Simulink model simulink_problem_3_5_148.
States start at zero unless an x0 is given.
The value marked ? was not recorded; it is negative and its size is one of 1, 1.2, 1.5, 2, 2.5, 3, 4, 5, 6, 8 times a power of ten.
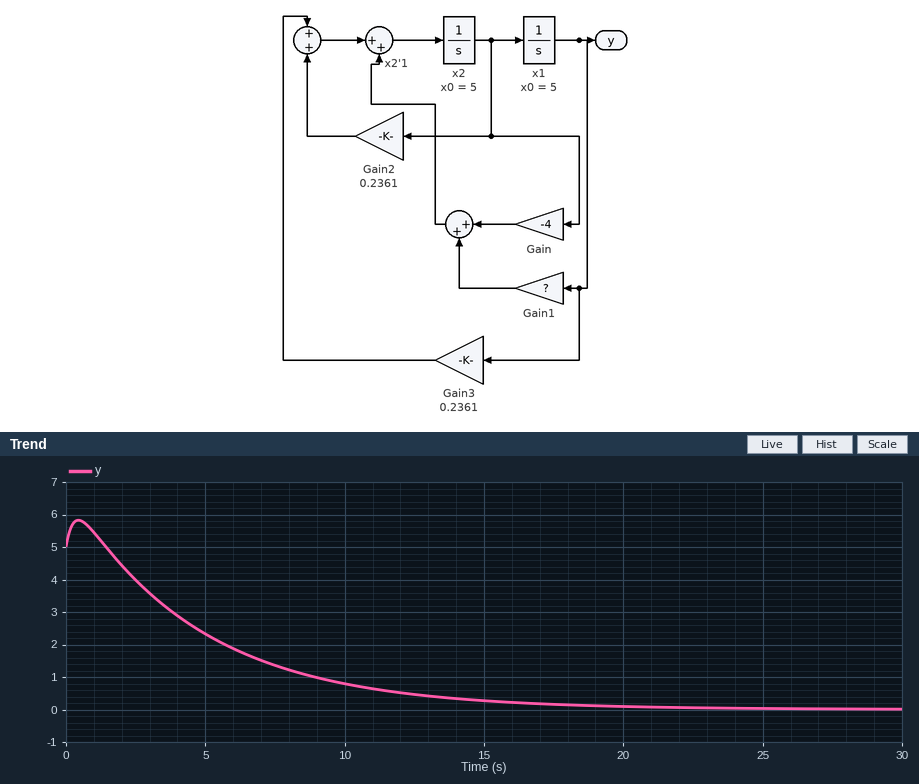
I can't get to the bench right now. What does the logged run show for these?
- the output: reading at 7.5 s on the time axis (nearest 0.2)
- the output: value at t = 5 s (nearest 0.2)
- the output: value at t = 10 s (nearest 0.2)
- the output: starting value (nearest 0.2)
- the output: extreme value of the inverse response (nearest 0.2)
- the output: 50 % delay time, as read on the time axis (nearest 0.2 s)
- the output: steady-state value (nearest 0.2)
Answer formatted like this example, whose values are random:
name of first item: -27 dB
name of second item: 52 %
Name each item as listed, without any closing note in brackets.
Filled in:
the output: reading at 7.5 s on the time axis: 1.4
the output: value at t = 5 s: 2.4
the output: value at t = 10 s: 0.8
the output: starting value: 5.0
the output: extreme value of the inverse response: 5.8
the output: 50 % delay time, as read on the time axis: 4.6 s
the output: steady-state value: 0.0
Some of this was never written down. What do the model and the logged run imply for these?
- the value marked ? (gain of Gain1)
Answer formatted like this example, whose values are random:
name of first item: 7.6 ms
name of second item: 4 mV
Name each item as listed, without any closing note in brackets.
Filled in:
the value marked ?: -1
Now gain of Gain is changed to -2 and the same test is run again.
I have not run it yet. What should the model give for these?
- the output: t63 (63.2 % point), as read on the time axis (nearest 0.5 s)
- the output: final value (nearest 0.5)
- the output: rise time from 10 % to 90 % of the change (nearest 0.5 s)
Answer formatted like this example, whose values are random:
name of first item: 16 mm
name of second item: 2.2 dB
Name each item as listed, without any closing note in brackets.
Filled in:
the output: t63 (63.2 % point), as read on the time axis: 3.5 s
the output: final value: 0.0
the output: rise time from 10 % to 90 % of the change: 3.5 s
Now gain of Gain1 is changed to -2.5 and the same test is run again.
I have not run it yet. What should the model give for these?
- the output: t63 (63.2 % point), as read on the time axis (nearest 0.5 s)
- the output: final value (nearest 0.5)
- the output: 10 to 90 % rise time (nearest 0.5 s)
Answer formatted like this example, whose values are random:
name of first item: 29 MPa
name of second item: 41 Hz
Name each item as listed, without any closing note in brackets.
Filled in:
the output: t63 (63.2 % point), as read on the time axis: 2.0 s
the output: final value: 0.0
the output: 10 to 90 % rise time: 3.0 s
